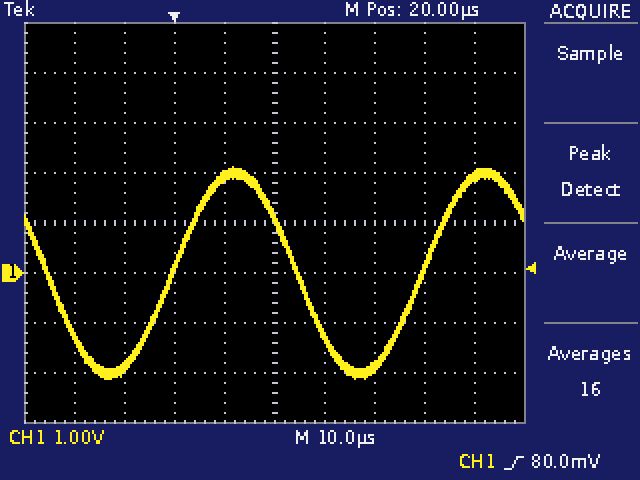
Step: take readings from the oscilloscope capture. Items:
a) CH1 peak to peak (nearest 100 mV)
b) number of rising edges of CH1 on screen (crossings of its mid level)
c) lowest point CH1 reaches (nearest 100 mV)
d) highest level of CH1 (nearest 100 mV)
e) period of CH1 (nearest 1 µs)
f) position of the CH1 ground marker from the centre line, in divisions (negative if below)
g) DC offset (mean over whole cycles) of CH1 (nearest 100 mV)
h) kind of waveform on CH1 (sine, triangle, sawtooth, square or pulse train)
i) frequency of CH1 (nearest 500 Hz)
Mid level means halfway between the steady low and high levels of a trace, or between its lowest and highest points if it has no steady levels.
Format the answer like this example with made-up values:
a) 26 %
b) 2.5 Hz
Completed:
a) 4.2 V
b) 2
c) -2.1 V
d) 2.1 V
e) 50 µs
f) -1.0 div
g) 0.0 V
h) sine
i) 20.0 kHz
